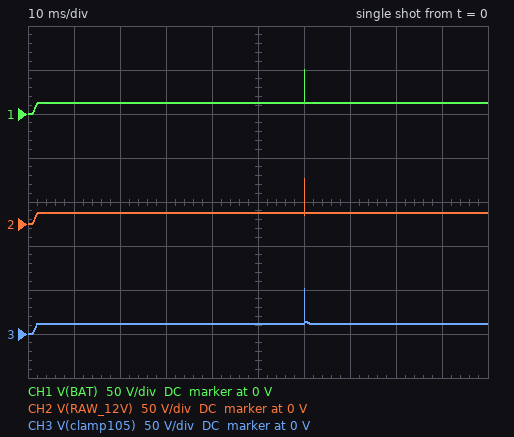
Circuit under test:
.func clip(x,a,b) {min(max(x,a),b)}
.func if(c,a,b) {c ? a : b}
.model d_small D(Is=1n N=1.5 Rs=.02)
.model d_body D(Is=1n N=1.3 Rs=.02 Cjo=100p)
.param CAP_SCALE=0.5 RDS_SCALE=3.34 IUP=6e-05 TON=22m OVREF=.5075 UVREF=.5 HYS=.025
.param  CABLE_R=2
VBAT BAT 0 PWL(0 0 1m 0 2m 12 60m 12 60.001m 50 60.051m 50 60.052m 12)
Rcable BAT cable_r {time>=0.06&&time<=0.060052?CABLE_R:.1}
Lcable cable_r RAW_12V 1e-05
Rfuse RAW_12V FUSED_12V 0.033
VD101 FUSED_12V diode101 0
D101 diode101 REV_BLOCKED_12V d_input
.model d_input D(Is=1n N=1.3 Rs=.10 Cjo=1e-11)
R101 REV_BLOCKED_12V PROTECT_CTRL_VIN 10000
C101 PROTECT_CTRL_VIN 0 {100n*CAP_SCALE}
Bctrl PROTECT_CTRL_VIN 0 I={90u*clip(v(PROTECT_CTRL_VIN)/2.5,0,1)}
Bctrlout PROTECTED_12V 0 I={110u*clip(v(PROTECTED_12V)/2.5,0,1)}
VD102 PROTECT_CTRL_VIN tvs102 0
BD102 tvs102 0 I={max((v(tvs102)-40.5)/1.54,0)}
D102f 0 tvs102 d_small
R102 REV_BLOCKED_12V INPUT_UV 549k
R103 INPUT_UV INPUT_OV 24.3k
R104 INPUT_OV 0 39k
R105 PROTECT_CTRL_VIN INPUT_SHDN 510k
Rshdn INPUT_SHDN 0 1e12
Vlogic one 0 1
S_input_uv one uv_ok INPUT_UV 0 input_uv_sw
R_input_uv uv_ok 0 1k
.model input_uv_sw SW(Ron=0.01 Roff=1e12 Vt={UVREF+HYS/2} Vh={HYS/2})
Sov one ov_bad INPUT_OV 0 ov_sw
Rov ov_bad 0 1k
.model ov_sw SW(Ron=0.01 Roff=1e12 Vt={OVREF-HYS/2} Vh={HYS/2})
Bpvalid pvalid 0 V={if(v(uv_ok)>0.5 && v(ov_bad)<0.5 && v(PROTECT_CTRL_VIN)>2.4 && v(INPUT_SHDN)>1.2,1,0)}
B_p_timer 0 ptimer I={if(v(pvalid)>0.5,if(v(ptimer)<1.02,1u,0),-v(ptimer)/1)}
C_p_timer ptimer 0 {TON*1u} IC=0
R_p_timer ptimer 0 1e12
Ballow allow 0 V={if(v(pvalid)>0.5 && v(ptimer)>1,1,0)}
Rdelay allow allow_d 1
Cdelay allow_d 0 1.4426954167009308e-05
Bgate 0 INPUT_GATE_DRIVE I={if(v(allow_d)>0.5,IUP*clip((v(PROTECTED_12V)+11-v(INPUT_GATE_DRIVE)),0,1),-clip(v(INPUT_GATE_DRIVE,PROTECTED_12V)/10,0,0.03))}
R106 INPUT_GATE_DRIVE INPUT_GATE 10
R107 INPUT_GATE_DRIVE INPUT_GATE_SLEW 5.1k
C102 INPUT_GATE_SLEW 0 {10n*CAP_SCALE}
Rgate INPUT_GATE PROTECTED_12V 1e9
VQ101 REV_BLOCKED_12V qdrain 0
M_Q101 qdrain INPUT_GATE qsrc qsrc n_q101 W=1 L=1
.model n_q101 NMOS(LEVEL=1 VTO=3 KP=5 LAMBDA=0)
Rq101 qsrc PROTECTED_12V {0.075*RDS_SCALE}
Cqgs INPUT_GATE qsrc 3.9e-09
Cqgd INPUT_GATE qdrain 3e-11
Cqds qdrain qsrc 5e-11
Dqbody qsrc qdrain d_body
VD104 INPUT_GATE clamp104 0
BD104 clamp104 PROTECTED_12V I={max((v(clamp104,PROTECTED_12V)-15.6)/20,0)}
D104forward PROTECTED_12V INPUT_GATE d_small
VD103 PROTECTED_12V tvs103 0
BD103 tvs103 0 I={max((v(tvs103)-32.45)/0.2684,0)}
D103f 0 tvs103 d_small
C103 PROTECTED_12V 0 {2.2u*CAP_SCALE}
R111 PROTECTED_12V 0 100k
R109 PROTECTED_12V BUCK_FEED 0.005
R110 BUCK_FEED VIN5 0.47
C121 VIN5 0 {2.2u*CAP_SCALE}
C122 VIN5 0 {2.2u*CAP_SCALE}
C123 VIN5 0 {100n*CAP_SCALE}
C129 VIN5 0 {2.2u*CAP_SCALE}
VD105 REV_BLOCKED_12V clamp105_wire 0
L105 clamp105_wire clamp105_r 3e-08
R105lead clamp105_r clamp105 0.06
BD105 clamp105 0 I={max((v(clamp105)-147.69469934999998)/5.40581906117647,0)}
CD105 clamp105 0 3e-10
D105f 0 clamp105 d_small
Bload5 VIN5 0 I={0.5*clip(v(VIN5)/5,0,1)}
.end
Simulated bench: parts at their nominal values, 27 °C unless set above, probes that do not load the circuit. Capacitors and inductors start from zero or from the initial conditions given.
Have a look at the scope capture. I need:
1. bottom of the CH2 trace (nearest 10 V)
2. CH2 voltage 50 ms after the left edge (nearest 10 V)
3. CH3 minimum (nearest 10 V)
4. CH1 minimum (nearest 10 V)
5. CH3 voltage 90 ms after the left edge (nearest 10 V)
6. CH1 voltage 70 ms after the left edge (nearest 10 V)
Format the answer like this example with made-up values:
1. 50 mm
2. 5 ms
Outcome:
1. 0 V
2. 10 V
3. 0 V
4. 0 V
5. 10 V
6. 10 V
